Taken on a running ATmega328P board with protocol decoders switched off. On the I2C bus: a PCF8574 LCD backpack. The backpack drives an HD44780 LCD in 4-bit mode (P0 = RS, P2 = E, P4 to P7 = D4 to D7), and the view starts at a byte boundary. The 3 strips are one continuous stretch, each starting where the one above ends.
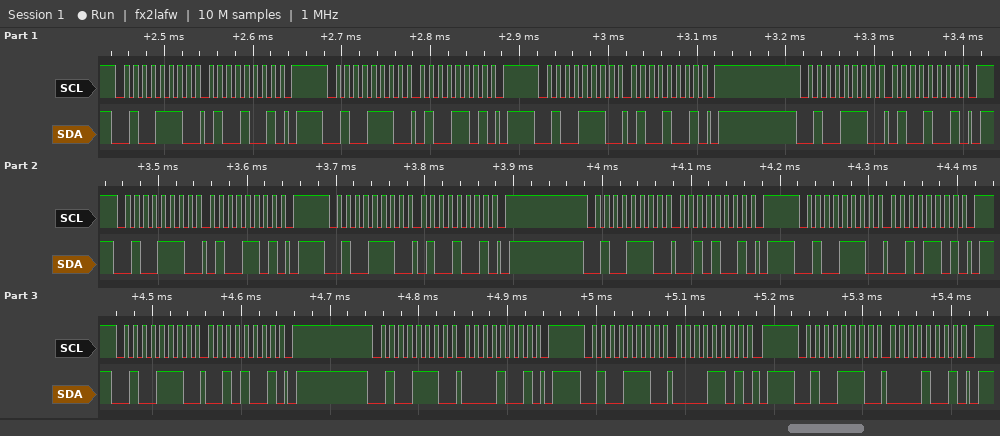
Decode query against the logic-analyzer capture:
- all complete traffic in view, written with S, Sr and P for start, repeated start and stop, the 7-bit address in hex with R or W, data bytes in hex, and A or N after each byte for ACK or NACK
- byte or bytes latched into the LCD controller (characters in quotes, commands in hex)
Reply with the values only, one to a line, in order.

S 27W A 49 A P S 27W A 4D A P S 27W A 49 A P S 27W A 49 A P S 27W A 4D A P S 27W A 49 A P S 27W A 29 A P S 27W A 2D A P S 27W A 29 A P S 27W A 09 A P S 27W A 0D A P S 27W A 09 A P
'D' ' '
